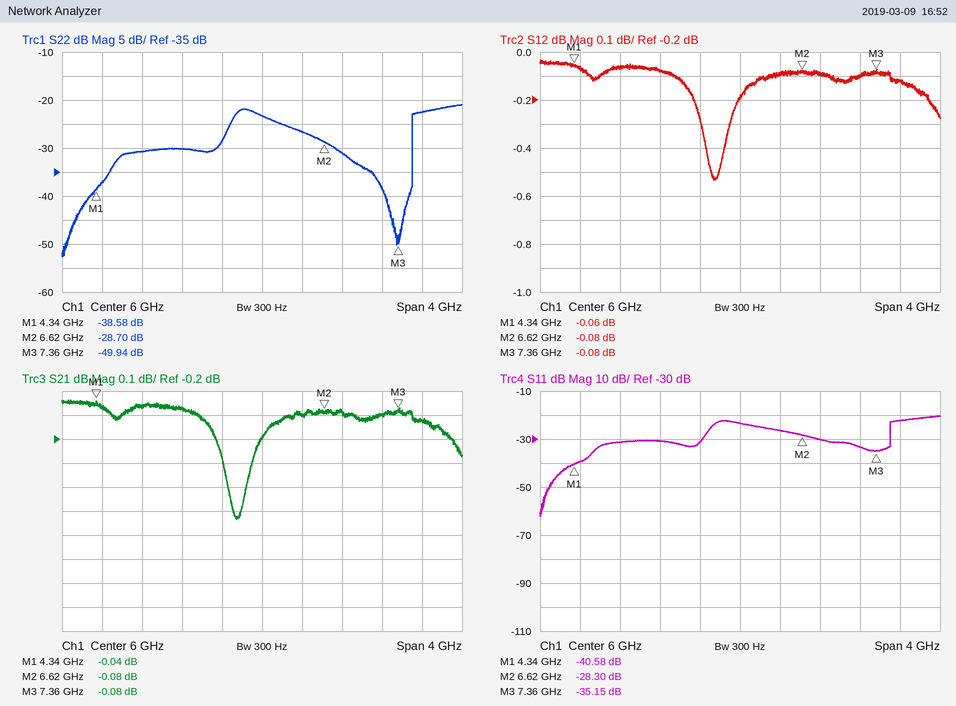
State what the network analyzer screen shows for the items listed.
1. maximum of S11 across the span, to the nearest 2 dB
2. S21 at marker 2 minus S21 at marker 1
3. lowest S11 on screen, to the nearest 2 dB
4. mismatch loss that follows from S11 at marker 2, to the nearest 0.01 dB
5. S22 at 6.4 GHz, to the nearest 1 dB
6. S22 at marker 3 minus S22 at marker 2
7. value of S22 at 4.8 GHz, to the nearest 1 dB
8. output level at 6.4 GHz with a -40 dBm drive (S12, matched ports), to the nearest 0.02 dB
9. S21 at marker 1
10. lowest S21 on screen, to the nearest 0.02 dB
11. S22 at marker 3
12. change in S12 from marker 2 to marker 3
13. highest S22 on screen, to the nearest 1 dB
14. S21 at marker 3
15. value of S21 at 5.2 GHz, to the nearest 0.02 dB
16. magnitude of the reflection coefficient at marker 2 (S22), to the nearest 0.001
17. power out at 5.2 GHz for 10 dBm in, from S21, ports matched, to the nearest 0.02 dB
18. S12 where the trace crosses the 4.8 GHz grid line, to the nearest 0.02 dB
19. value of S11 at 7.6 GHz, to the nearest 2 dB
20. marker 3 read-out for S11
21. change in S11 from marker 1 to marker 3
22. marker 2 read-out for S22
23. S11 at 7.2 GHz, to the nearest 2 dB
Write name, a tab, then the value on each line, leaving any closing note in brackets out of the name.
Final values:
maximum of S11 across the span, to the nearest 2 dB	-20 dB
S21 at marker 2 minus S21 at marker 1	-0.04 dB
lowest S11 on screen, to the nearest 2 dB	-62 dB
mismatch loss that follows from S11 at marker 2, to the nearest 0.01 dB	0.01 dB
S22 at 6.4 GHz, to the nearest 1 dB	-27 dB
S22 at marker 3 minus S22 at marker 2	-21.24 dB
value of S22 at 4.8 GHz, to the nearest 1 dB	-31 dB
output level at 6.4 GHz with a -40 dBm drive (S12, matched ports), to the nearest 0.02 dB	-40.10 dBm
S21 at marker 1	-0.04 dB
lowest S21 on screen, to the nearest 0.02 dB	-0.54 dB
S22 at marker 3	-49.94 dB
change in S12 from marker 2 to marker 3	0.00 dB
highest S22 on screen, to the nearest 1 dB	-21 dB
S21 at marker 3	-0.08 dB
value of S21 at 5.2 GHz, to the nearest 0.02 dB	-0.08 dB
magnitude of the reflection coefficient at marker 2 (S22), to the nearest 0.001	0.037
power out at 5.2 GHz for 10 dBm in, from S21, ports matched, to the nearest 0.02 dB	9.92 dBm
S12 where the trace crosses the 4.8 GHz grid line, to the nearest 0.02 dB	-0.06 dB
value of S11 at 7.6 GHz, to the nearest 2 dB	-22 dB
marker 3 read-out for S11	-35.15 dB
change in S11 from marker 1 to marker 3	5.43 dB
marker 2 read-out for S22	-28.70 dB
S11 at 7.2 GHz, to the nearest 2 dB	-34 dB
